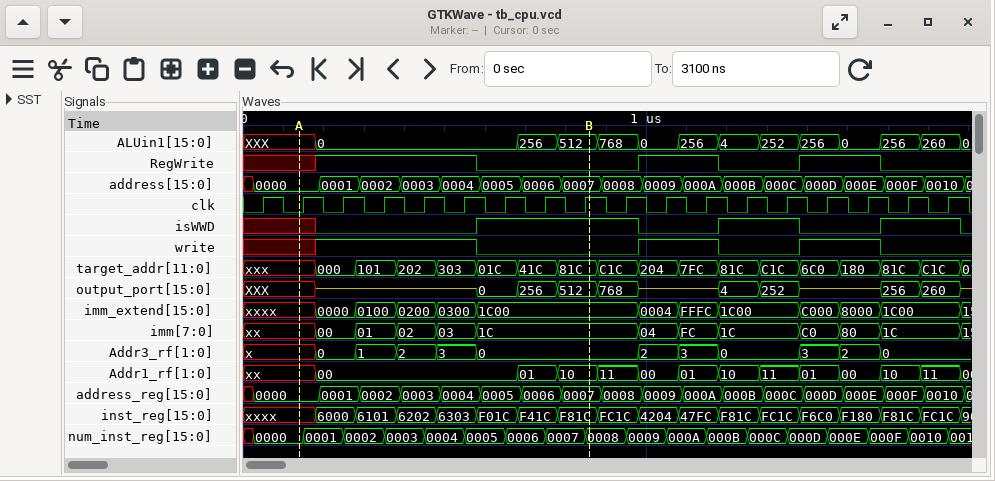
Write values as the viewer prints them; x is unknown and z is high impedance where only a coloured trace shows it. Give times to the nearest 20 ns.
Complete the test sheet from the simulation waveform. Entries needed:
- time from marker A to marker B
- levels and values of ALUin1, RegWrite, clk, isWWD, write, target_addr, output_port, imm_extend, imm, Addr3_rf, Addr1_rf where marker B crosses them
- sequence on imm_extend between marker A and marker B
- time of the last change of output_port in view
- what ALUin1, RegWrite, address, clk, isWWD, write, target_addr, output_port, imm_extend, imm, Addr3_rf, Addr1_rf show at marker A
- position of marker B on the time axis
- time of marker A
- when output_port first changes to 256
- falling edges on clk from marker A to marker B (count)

720 ns
ALUin1=512, RegWrite=0, clk=1, isWWD=1, write=0, target_addr=81C, output_port=512, imm_extend=1C00, imm=1C, Addr3_rf=0, Addr1_rf=10
xxxx, 0000, 0100, 0200, 0300, 1C00
1780 ns
ALUin1=XXX, RegWrite=x, address=0000, clk=0, isWWD=x, write=x, target_addr=xxx, output_port=XXX, imm_extend=xxxx, imm=xx, Addr3_rf=x, Addr1_rf=xx
860 ns
140 ns
680 ns
7
